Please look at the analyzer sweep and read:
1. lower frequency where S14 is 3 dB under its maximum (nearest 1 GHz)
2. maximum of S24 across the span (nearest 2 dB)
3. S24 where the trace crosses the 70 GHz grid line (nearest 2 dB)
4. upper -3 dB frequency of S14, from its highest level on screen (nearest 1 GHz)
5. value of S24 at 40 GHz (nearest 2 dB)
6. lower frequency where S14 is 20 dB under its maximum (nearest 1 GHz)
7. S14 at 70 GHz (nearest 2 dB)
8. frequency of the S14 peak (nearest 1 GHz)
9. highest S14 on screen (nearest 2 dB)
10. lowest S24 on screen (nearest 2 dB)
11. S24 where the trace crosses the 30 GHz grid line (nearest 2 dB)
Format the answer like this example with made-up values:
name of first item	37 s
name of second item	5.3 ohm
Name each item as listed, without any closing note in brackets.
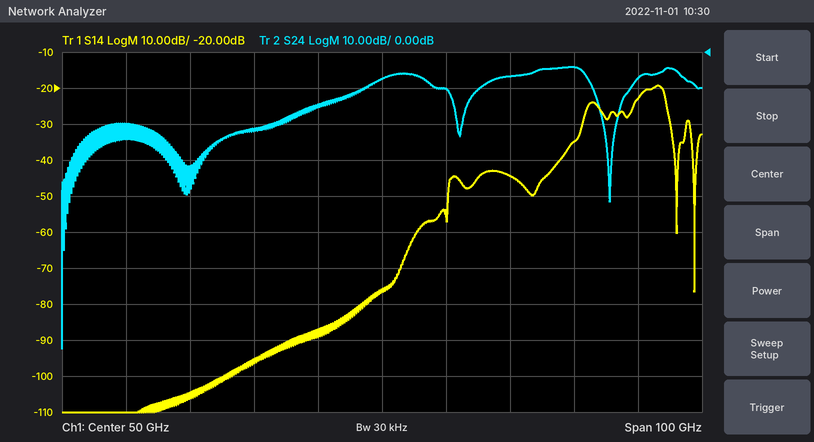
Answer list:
lower frequency where S14 is 3 dB under its maximum	90 GHz
maximum of S24 across the span	-4 dB
S24 where the trace crosses the 70 GHz grid line	-6 dB
upper -3 dB frequency of S14, from its highest level on screen	94 GHz
value of S24 at 40 GHz	-14 dB
lower frequency where S14 is 20 dB under its maximum	78 GHz
S14 at 70 GHz	-44 dB
frequency of the S14 peak	93 GHz
highest S14 on screen	-20 dB
lowest S24 on screen	-82 dB
S24 where the trace crosses the 30 GHz grid line	-22 dB
